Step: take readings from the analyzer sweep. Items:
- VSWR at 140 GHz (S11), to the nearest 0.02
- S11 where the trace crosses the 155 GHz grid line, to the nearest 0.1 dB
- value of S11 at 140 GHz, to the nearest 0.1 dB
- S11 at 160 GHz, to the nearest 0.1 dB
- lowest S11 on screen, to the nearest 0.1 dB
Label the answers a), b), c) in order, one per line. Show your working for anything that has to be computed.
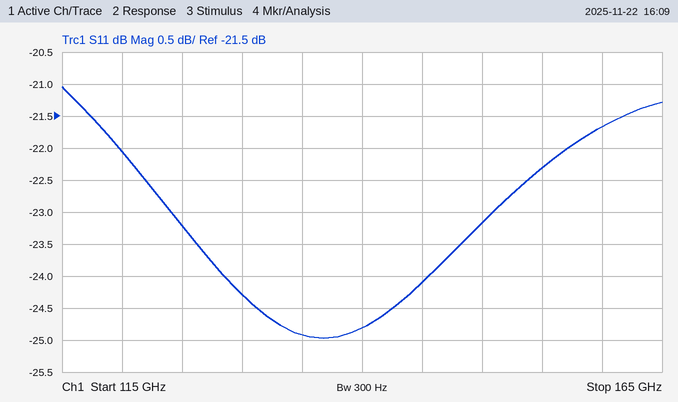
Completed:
a) |Γ| = 10^(-24.8/20) = 0.0575; VSWR = (1 + 0.0575)/(1 − 0.0575) ≈ 1.12
b) -22.3 dB
c) -24.8 dB
d) -21.7 dB
e) -25.0 dB
